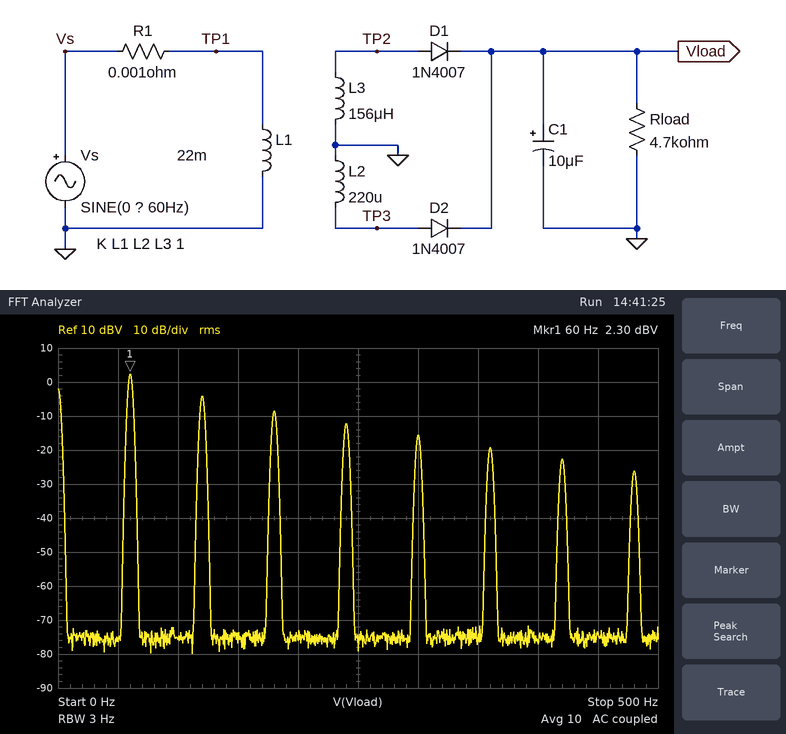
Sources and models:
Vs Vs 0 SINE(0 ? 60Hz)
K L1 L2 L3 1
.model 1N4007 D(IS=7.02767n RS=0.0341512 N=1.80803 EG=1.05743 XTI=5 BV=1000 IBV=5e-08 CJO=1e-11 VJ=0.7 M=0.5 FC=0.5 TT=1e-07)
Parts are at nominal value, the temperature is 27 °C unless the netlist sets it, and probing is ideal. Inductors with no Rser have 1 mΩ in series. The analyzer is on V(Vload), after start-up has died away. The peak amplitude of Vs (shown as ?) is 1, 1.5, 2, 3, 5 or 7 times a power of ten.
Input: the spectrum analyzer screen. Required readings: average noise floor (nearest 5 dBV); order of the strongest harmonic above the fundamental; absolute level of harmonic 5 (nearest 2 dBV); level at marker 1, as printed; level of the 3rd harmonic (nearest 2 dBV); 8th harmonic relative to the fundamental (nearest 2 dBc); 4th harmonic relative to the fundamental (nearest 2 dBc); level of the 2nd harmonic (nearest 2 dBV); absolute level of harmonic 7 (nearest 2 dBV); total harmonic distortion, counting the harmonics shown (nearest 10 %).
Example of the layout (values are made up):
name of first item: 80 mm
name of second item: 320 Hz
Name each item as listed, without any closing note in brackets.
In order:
average noise floor: -75 dBV
order of the strongest harmonic above the fundamental: 2
absolute level of harmonic 5: -16 dBV
level at marker 1, as printed: 2.30 dBV
level of the 3rd harmonic: -8 dBV
8th harmonic relative to the fundamental: -28 dBc
4th harmonic relative to the fundamental: -14 dBc
level of the 2nd harmonic: -4 dBV
absolute level of harmonic 7: -22 dBV
total harmonic distortion, counting the harmonics shown: 60 %
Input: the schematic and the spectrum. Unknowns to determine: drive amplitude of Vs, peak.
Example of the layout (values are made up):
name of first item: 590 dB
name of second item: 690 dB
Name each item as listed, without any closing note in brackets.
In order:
drive amplitude of Vs, peak: 200 V
